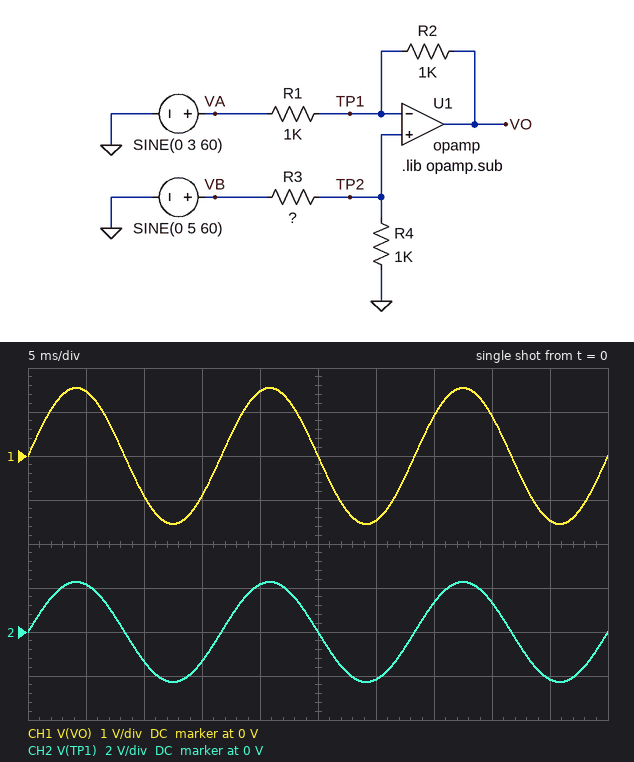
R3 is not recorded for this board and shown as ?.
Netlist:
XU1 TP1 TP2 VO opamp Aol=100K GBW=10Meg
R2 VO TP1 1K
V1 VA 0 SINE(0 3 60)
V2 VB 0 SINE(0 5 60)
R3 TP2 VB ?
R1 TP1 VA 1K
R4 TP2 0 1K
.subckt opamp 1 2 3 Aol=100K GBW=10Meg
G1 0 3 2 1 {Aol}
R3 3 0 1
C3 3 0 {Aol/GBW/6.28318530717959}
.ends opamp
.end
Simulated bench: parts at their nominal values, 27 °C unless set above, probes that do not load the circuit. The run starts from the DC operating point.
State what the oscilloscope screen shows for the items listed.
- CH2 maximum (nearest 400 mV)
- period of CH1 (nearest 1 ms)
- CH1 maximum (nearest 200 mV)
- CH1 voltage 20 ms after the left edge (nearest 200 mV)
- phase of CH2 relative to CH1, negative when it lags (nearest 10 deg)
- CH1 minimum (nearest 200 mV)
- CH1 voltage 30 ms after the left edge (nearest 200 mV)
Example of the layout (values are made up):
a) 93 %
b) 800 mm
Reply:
a) 2.4 V
b) 17 ms
c) 1.6 V
d) 1.4 V
e) 0 deg
f) -1.6 V
g) -1.4 V
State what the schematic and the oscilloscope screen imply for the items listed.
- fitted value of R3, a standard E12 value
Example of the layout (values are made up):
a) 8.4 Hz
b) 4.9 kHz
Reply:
a) 1.2 kΩ
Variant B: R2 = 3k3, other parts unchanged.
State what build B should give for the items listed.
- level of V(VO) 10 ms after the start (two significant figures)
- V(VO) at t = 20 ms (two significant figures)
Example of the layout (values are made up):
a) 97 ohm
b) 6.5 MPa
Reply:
a) 75 mV
b) -120 mV
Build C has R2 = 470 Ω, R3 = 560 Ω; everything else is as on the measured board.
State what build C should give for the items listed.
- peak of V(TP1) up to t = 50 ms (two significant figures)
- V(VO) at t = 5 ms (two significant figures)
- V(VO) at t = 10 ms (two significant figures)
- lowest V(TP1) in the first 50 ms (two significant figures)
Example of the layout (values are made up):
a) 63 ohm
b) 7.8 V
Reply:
a) 3.2 V
b) 3.1 V
c) -1.9 V
d) -3.2 V
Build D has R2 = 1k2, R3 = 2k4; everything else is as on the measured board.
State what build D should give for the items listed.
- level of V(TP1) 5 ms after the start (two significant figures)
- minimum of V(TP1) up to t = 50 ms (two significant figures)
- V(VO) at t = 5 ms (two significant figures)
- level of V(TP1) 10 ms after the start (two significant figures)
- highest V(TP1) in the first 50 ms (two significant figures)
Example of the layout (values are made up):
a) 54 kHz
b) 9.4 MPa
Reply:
a) 1.4 V
b) -1.5 V
c) -350 mV
d) -860 mV
e) 1.5 V
